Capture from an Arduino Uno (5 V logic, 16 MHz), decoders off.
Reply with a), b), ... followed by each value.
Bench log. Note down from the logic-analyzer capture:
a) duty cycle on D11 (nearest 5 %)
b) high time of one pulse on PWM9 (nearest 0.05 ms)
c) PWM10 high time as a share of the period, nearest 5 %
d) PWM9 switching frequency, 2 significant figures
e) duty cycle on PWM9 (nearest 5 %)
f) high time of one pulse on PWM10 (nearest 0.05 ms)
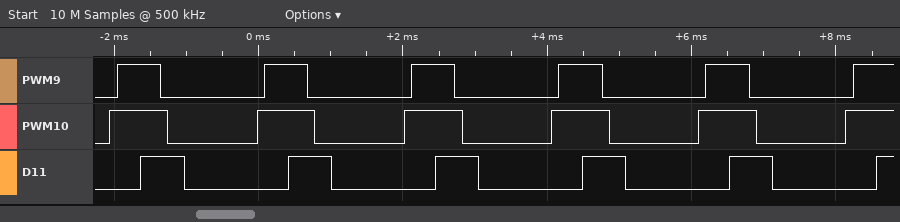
a) 30 %
b) 0.60 ms
c) 40 %
d) 490 Hz
e) 30 %
f) 0.80 ms
